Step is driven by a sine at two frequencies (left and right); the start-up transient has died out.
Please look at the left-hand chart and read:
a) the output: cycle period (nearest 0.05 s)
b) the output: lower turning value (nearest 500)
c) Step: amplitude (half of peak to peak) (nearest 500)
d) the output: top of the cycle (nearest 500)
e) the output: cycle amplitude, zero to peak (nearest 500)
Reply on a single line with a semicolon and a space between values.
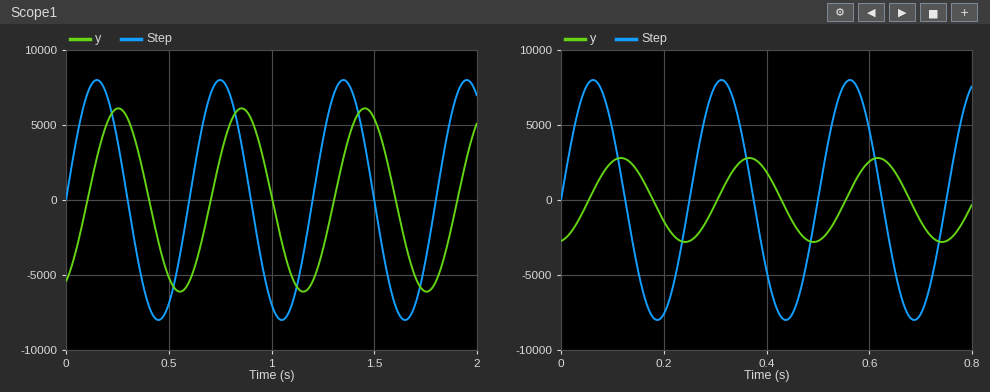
0.60 s; -6000; 8000; 6000; 6000
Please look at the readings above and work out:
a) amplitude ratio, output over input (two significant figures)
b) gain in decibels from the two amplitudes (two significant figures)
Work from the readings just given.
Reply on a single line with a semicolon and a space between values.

0.75; -2.5 dB
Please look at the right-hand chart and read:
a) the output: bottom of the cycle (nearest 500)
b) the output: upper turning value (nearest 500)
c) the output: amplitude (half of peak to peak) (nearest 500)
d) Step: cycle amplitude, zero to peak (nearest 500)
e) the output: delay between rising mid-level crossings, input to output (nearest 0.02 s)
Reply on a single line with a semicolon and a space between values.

-3000; 3000; 3000; 8000; 0.06 s
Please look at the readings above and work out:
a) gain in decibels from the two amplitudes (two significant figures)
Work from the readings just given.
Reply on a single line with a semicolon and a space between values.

-8.5 dB
